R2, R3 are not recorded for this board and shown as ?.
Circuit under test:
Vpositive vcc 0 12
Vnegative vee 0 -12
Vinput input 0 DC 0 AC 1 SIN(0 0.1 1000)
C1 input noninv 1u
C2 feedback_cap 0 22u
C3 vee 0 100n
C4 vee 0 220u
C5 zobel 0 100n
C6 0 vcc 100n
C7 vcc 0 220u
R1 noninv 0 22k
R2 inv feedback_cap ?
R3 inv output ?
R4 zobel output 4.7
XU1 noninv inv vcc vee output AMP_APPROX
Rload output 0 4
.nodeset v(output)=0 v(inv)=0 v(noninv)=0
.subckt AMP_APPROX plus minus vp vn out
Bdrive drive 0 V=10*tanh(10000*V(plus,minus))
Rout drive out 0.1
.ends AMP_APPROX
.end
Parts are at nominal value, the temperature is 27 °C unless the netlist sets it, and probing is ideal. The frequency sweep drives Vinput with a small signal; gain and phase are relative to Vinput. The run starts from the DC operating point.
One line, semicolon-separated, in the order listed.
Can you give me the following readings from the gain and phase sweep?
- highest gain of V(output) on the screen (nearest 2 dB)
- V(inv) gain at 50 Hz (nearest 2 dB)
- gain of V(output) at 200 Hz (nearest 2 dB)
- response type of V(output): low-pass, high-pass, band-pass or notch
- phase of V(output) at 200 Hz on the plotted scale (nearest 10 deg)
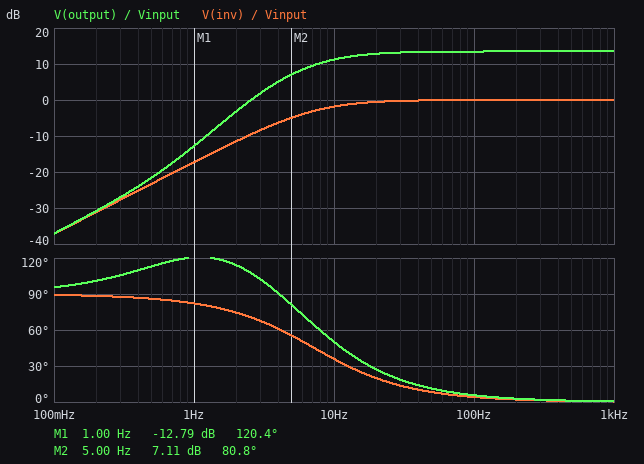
14 dB; 0 dB; 14 dB; high-pass; 0 deg
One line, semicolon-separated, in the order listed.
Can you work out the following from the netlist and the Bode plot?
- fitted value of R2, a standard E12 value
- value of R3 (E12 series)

2.2 kΩ; 8.2 kΩ
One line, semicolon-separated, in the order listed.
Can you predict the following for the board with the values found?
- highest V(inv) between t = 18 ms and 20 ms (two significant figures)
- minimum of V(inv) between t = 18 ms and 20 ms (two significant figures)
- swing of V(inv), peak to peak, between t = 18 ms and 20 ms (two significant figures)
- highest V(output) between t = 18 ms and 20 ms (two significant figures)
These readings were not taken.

100 mV; -100 mV; 200 mV; 470 mV
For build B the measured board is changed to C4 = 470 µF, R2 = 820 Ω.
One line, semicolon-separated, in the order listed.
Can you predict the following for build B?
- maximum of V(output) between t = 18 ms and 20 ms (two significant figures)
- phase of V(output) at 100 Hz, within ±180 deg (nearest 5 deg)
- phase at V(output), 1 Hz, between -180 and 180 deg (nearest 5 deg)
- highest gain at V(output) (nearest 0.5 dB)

1.1 V; 10 deg; 125 deg; 21.0 dB
